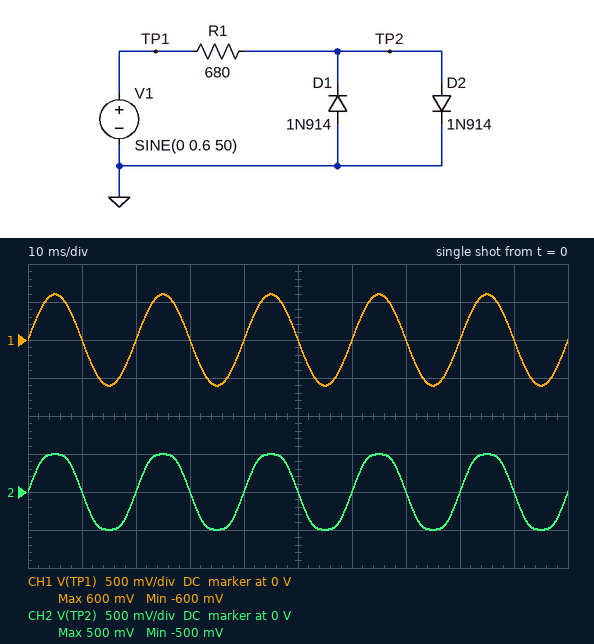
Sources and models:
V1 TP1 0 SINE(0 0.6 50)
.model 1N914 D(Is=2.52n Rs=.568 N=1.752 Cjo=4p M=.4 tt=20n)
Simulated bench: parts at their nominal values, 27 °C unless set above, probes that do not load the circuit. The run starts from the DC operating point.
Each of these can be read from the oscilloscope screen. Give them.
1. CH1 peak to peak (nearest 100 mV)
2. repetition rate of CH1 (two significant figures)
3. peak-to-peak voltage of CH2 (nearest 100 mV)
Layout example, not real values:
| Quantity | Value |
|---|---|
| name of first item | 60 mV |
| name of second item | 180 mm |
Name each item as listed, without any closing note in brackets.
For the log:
| Quantity | Value |
|---|---|
| CH1 peak to peak | 1.2 V |
| repetition rate of CH1 | 50 Hz |
| peak-to-peak voltage of CH2 | 1.0 V |
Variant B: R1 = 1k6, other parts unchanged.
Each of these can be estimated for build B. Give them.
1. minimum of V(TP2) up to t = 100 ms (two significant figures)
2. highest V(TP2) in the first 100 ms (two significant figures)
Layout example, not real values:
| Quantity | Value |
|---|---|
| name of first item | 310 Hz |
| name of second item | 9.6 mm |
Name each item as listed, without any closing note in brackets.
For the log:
| Quantity | Value |
|---|---|
| minimum of V(TP2) up to t = 100 ms | -470 mV |
| highest V(TP2) in the first 100 ms | 470 mV |
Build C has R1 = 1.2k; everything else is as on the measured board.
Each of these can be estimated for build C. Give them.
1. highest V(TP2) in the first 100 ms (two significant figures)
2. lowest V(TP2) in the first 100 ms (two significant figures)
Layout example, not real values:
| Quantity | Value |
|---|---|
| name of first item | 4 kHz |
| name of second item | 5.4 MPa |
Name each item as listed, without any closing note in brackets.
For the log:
| Quantity | Value |
|---|---|
| highest V(TP2) in the first 100 ms | 480 mV |
| lowest V(TP2) in the first 100 ms | -480 mV |
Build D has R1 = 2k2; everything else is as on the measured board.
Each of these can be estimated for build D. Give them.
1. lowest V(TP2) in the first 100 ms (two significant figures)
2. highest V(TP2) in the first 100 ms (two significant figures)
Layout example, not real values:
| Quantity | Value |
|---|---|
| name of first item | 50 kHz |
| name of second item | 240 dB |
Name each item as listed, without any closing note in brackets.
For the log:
| Quantity | Value |
|---|---|
| lowest V(TP2) in the first 100 ms | -460 mV |
| highest V(TP2) in the first 100 ms | 460 mV |
